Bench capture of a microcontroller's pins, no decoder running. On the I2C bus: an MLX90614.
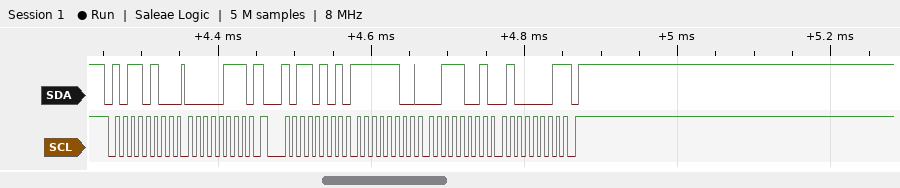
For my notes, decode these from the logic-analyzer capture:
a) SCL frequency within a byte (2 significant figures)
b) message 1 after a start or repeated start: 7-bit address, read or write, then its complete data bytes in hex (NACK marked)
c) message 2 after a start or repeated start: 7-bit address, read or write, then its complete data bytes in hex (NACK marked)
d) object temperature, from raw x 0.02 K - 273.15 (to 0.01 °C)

100 kHz
0x5A write: 07
0x5A read: FC 39 41 NACK
23.73 °C
